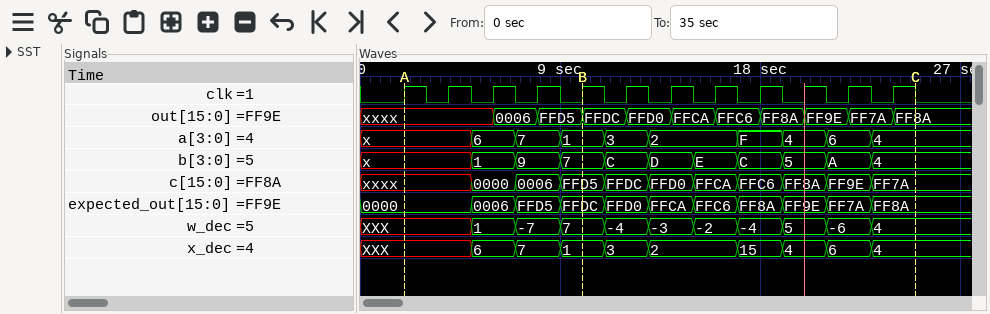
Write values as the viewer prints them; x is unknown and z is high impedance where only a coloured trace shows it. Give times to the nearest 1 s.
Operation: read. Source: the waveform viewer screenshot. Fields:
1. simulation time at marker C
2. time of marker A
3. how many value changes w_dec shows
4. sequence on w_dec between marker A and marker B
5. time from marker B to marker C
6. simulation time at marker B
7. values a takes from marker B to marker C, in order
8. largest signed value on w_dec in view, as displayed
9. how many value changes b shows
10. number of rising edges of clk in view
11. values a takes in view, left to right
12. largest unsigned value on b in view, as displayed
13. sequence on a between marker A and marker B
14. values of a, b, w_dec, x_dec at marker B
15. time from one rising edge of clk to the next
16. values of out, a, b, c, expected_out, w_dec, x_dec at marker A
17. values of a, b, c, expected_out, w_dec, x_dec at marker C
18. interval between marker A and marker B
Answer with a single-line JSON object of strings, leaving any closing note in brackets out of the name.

{"simulation time at marker C": "25 s", "time of marker A": "2 s", "how many value changes w_dec shows": "10", "sequence on w_dec between marker A and marker B": "XXX, 1, -7, 7", "time from marker B to marker C": "15 s", "simulation time at marker B": "10 s", "values a takes from marker B to marker C, in order": "1, 3, 2, F, 4, 6, 4", "largest signed value on w_dec in view, as displayed": "7", "how many value changes b shows": "10", "number of rising edges of clk in view": "12", "values a takes in view, left to right": "x, 6, 7, 1, 3, 2, F, 4, 6, 4", "largest unsigned value on b in view, as displayed": "E", "sequence on a between marker A and marker B": "x, 6, 7, 1", "values of a, b, w_dec, x_dec at marker B": "a=1, b=7, w_dec=7, x_dec=1", "time from one rising edge of clk to the next": "2 s", "values of out, a, b, c, expected_out, w_dec, x_dec at marker A": "out=xxxx, a=x, b=x, c=xxxx, expected_out=0000, w_dec=XXX, x_dec=XXX", "values of a, b, c, expected_out, w_dec, x_dec at marker C": "a=4, b=4, c=FF7A, expected_out=FF8A, w_dec=4, x_dec=4", "interval between marker A and marker B": "8 s"}
